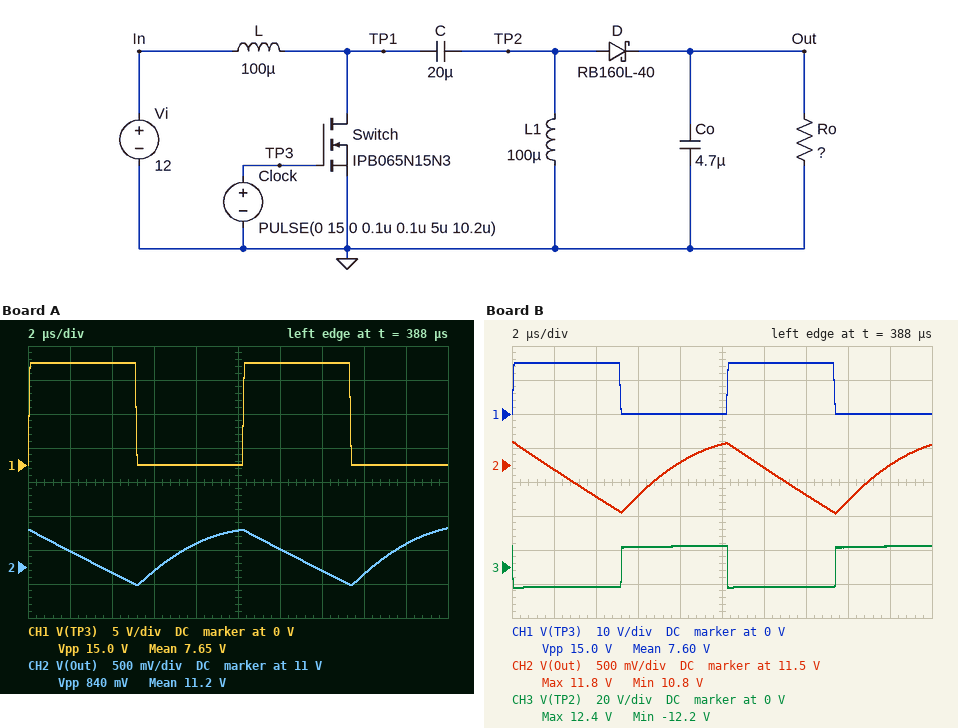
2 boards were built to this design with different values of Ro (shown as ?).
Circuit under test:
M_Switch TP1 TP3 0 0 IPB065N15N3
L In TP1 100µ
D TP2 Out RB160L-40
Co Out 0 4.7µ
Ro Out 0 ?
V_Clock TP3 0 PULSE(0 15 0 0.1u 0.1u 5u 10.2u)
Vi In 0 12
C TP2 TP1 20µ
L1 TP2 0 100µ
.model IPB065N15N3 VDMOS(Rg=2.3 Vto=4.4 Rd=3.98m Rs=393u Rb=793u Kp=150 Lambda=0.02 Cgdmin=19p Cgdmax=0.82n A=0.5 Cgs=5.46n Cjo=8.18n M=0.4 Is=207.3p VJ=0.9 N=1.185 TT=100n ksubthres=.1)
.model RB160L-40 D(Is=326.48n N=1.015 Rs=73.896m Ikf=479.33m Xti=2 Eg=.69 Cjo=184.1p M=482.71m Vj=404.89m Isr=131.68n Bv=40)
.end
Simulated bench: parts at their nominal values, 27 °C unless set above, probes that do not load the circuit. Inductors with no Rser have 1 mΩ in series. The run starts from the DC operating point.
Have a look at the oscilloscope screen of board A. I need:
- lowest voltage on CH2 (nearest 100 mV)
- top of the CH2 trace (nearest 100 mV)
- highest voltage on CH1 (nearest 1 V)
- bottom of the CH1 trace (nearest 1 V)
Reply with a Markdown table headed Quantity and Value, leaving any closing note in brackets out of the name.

| Quantity | Value |
|---|---|
| lowest voltage on CH2 | 10.7 V |
| top of the CH2 trace | 11.6 V |
| highest voltage on CH1 | 15 V |
| bottom of the CH1 trace | 0 V |
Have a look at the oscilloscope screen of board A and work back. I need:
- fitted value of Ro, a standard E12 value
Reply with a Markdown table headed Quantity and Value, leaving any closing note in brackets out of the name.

| Quantity | Value |
|---|---|
| fitted value of Ro, a standard E12 value | 15 Ω |
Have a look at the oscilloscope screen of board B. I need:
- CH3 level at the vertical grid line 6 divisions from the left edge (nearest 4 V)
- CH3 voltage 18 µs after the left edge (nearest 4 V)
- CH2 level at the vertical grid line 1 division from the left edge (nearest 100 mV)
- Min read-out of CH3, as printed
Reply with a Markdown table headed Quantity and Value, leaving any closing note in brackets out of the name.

| Quantity | Value |
|---|---|
| CH3 level at the vertical grid line 6 divisions from the left edge | -12 V |
| CH3 voltage 18 µs after the left edge | 12 V |
| CH2 level at the vertical grid line 1 division from the left edge | 11.4 V |
| Min read-out of CH3, as printed | -12.2 V |
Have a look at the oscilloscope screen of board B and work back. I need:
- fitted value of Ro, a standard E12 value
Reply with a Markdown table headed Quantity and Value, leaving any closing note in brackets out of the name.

| Quantity | Value |
|---|---|
| fitted value of Ro, a standard E12 value | 12 Ω |
